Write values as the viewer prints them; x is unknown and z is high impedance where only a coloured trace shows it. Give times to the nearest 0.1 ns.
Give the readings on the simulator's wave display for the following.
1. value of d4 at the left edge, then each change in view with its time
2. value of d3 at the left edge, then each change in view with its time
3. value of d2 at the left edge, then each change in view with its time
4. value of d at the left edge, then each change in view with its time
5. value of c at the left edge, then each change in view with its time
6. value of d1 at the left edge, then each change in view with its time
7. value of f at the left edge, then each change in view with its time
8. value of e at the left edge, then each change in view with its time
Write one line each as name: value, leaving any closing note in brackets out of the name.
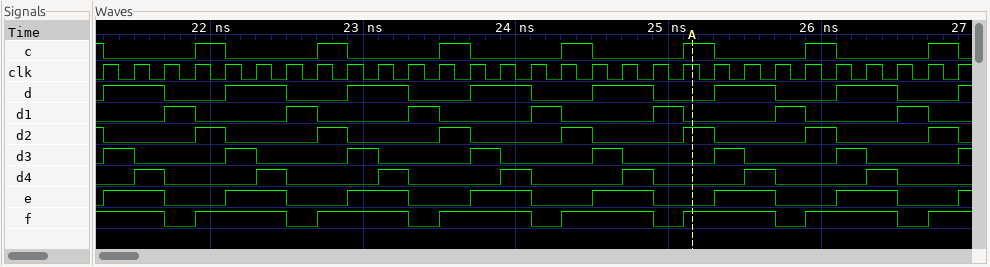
value of d4 at the left edge, then each change in view with its time: 0, 1 at 21.5 ns, 0 at 21.7 ns, 1 at 22.3 ns, 0 at 22.5 ns, 1 at 23.1 ns, 0 at 23.3 ns, 1 at 23.9 ns, 0 at 24.1 ns, 1 at 24.7 ns, 0 at 24.9 ns, 1 at 25.5 ns, 0 at 25.7 ns, 1 at 26.3 ns, 0 at 26.5 ns
value of d3 at the left edge, then each change in view with its time: 0, 1 at 21.3 ns, 0 at 21.5 ns, 1 at 22.1 ns, 0 at 22.3 ns, 1 at 22.9 ns, 0 at 23.1 ns, 1 at 23.7 ns, 0 at 23.9 ns, 1 at 24.5 ns, 0 at 24.7 ns, 1 at 25.3 ns, 0 at 25.5 ns, 1 at 26.1 ns, 0 at 26.3 ns, 1 at 26.9 ns
value of d2 at the left edge, then each change in view with its time: 1, 0 at 21.3 ns, 1 at 21.9 ns, 0 at 22.1 ns, 1 at 22.7 ns, 0 at 22.9 ns, 1 at 23.5 ns, 0 at 23.7 ns, 1 at 24.3 ns, 0 at 24.5 ns, 1 at 25.1 ns, 0 at 25.3 ns, 1 at 25.9 ns, 0 at 26.1 ns, 1 at 26.7 ns, 0 at 26.9 ns
value of d at the left edge, then each change in view with its time: 0, 1 at 21.3 ns, 0 at 21.7 ns, 1 at 22.1 ns, 0 at 22.5 ns, 1 at 22.9 ns, 0 at 23.3 ns, 1 at 23.7 ns, 0 at 24.1 ns, 1 at 24.5 ns, 0 at 24.9 ns, 1 at 25.3 ns, 0 at 25.7 ns, 1 at 26.1 ns, 0 at 26.5 ns, 1 at 26.9 ns
value of c at the left edge, then each change in view with its time: 1, 0 at 21.3 ns, 1 at 21.9 ns, 0 at 22.1 ns, 1 at 22.7 ns, 0 at 22.9 ns, 1 at 23.5 ns, 0 at 23.7 ns, 1 at 24.3 ns, 0 at 24.5 ns, 1 at 25.1 ns, 0 at 25.3 ns, 1 at 25.9 ns, 0 at 26.1 ns, 1 at 26.7 ns, 0 at 26.9 ns
value of d1 at the left edge, then each change in view with its time: 0, 1 at 21.7 ns, 0 at 21.9 ns, 1 at 22.5 ns, 0 at 22.7 ns, 1 at 23.3 ns, 0 at 23.5 ns, 1 at 24.1 ns, 0 at 24.3 ns, 1 at 24.9 ns, 0 at 25.1 ns, 1 at 25.7 ns, 0 at 25.9 ns, 1 at 26.5 ns, 0 at 26.7 ns
value of f at the left edge, then each change in view with its time: 1, 0 at 21.7 ns, 1 at 21.9 ns, 0 at 22.5 ns, 1 at 22.7 ns, 0 at 23.3 ns, 1 at 23.5 ns, 0 at 24.1 ns, 1 at 24.3 ns, 0 at 24.9 ns, 1 at 25.1 ns, 0 at 25.7 ns, 1 at 25.9 ns, 0 at 26.5 ns, 1 at 26.7 ns
value of e at the left edge, then each change in view with its time: 0, 1 at 21.3 ns, 0 at 21.7 ns, 1 at 22.1 ns, 0 at 22.5 ns, 1 at 22.9 ns, 0 at 23.3 ns, 1 at 23.7 ns, 0 at 24.1 ns, 1 at 24.5 ns, 0 at 24.9 ns, 1 at 25.3 ns, 0 at 25.7 ns, 1 at 26.1 ns, 0 at 26.5 ns, 1 at 26.9 ns
